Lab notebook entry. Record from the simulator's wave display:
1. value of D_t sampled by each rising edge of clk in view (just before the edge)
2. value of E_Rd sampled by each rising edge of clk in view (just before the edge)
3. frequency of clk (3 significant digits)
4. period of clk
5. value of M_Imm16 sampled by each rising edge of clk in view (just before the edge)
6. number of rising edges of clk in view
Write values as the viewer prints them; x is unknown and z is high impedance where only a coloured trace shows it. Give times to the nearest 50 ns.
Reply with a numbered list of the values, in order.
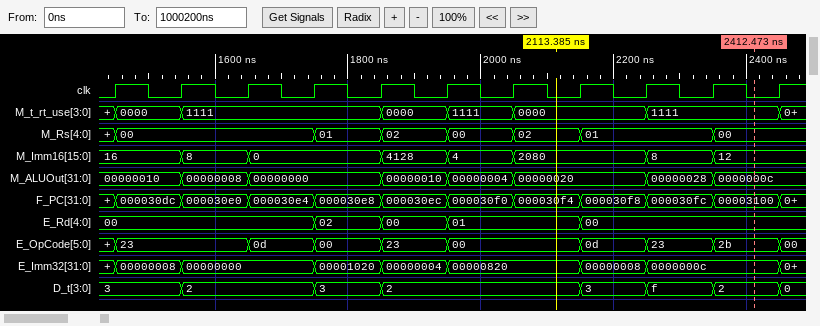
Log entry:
1. 3, 3, 2, 2, 3, 2, 2, 2, 3, f, 2
2. 00, 00, 00, 00, 02, 00, 01, 01, 00, 00, 00
3. 10.0 MHz
4. 100 ns
5. 16, 16, 8, 0, 0, 4128, 4, 2080, 2080, 8, 12
6. 11
